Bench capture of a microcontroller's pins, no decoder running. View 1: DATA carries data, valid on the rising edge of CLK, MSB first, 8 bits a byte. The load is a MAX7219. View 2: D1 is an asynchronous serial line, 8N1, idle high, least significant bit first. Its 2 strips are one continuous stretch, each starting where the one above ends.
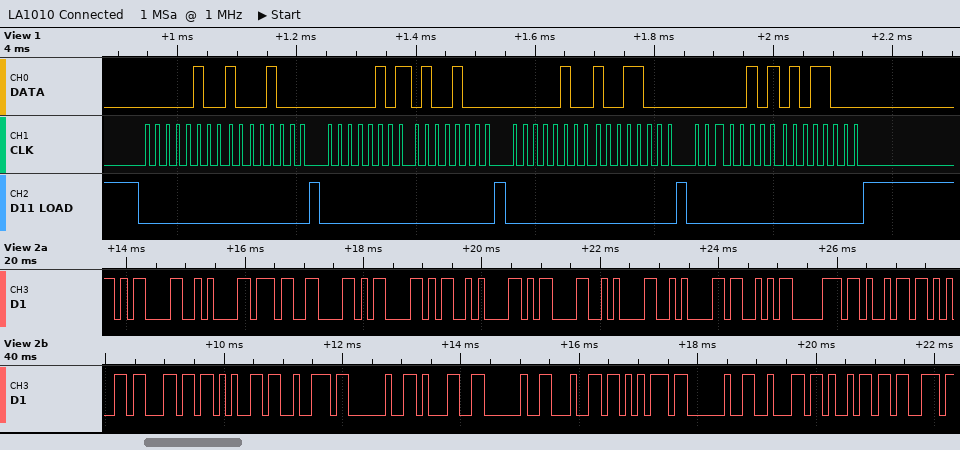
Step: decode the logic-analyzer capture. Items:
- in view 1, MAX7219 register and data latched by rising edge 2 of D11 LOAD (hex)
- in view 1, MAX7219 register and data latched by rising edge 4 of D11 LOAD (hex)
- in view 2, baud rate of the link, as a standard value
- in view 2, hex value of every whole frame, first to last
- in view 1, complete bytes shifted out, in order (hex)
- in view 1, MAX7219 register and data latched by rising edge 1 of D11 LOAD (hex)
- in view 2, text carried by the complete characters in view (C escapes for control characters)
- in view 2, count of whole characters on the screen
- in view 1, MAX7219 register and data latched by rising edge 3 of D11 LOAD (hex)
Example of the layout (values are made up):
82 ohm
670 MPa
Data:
register 0x5, data 0x48
register 0x5, data 0x58
9600 baud
0D 0A 37 58 58 0A 0D 0A 0A 53 70 69 65 6C 65 72 20 31 20 64 75 20 62 69 73
0x04 0x88 0x05 0x48 0x04 0x98 0x05 0x58
register 0x4, data 0x88
"\r\n7XX\n\r\n\nSpieler 1 du bis"
25
register 0x4, data 0x98
